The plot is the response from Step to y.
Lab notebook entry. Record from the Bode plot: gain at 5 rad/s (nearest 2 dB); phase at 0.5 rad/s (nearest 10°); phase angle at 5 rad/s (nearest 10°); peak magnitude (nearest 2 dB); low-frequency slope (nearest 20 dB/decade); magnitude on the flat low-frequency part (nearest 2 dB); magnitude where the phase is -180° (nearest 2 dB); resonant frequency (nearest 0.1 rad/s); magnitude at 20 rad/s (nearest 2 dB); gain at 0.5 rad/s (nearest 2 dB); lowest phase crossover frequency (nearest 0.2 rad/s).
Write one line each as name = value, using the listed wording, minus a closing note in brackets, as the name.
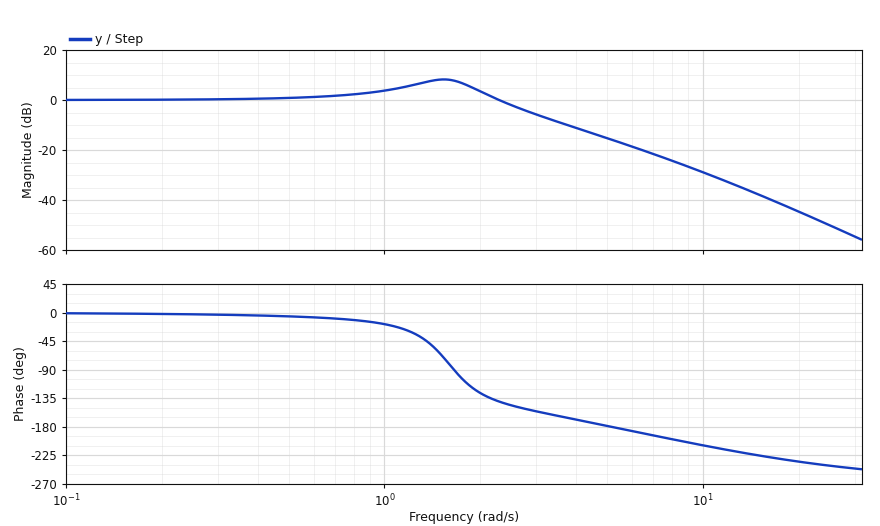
gain at 5 rad/s = -16 dB
phase at 0.5 rad/s = -10°
phase angle at 5 rad/s = -180°
peak magnitude = 8 dB
low-frequency slope = 0 dB/decade
magnitude on the flat low-frequency part = 0 dB
magnitude where the phase is -180° = -16 dB
resonant frequency = 1.5 rad/s
magnitude at 20 rad/s = -44 dB
gain at 0.5 rad/s = 0 dB
lowest phase crossover frequency = 5.2 rad/s
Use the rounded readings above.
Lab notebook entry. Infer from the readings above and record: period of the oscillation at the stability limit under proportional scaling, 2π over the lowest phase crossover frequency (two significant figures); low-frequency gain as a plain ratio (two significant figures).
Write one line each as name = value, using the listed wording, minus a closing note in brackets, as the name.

period of the oscillation at the stability limit under proportional scaling, 2π over the lowest phase crossover frequency = 1.2 s
low-frequency gain as a plain ratio = 1.0
